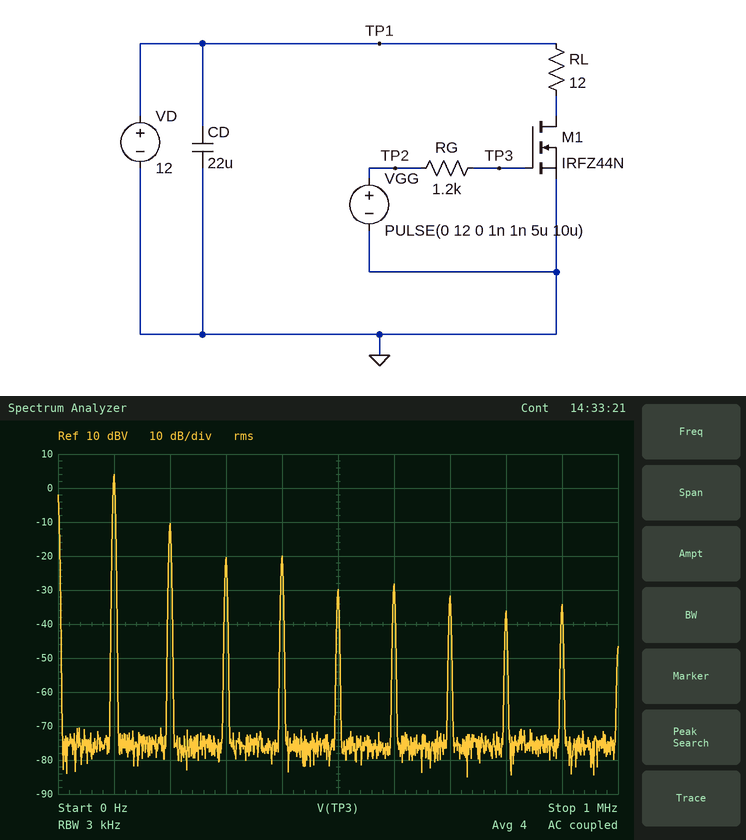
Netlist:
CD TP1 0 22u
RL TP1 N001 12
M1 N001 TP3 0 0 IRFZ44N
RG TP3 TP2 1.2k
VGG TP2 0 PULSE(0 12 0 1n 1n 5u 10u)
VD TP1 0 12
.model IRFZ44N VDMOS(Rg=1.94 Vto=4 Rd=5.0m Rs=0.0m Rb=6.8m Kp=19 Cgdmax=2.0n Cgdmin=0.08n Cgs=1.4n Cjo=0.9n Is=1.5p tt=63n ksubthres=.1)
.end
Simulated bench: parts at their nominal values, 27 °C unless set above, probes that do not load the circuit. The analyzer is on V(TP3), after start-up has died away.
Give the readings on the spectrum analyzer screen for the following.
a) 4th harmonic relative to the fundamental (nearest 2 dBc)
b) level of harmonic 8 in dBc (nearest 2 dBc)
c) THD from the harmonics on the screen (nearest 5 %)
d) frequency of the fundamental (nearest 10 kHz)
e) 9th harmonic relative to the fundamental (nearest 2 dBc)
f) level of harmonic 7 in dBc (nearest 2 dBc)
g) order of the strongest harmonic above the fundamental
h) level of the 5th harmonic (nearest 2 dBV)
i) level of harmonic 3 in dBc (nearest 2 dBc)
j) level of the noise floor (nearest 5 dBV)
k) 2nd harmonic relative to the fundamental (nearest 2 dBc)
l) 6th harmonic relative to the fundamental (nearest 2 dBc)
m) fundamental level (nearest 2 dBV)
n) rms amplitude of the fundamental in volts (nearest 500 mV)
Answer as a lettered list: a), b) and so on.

a) -24 dBc
b) -40 dBc
c) 20 %
d) 100 kHz
e) -38 dBc
f) -36 dBc
g) 2
h) -30 dBV
i) -24 dBc
j) -75 dBV
k) -14 dBc
l) -32 dBc
m) 4 dBV
n) 1.5 V
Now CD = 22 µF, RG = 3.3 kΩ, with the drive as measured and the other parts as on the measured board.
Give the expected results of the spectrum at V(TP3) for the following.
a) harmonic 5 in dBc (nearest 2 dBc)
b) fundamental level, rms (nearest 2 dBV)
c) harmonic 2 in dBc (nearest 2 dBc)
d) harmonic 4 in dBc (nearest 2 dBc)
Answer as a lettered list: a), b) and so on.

a) -28 dBc
b) -2 dBV
c) -48 dBc
d) -56 dBc
